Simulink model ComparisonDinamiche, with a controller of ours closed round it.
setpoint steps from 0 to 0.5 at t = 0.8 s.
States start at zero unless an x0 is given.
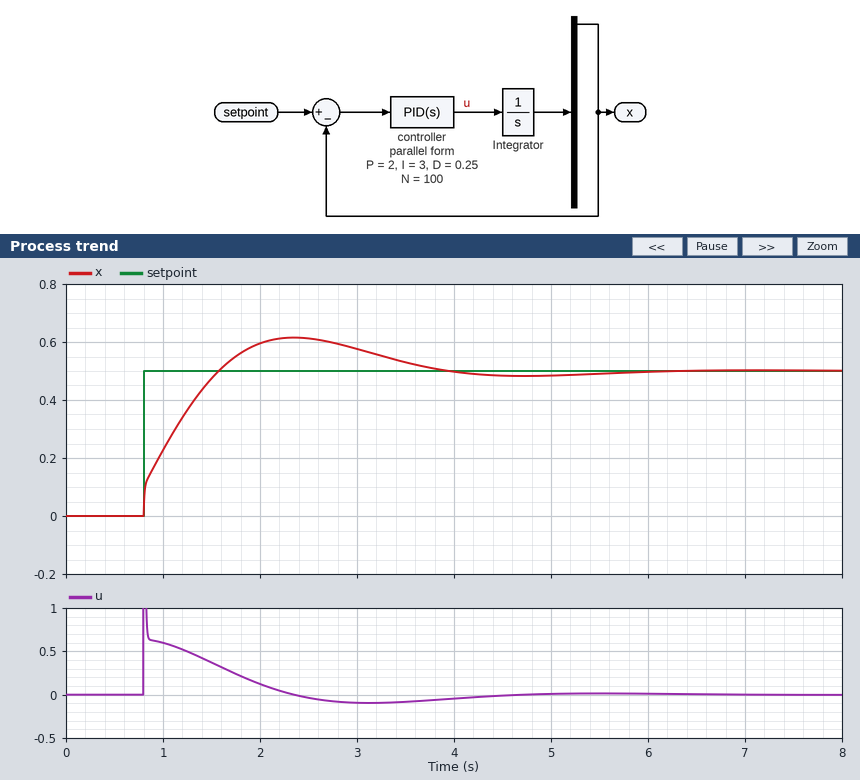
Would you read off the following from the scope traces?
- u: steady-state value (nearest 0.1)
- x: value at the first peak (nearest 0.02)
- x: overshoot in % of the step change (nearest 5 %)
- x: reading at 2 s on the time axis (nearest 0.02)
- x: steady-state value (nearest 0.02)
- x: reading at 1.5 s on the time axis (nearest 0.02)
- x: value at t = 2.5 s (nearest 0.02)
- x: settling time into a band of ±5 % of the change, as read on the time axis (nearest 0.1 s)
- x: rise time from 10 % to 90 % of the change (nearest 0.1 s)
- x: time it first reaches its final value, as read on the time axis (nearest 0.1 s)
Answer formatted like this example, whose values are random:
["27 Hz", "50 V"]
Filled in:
["0.0", "0.62", "25 %", "0.60", "0.50", "0.48", "0.62", "3.6 s", "0.6 s", "1.6 s"]
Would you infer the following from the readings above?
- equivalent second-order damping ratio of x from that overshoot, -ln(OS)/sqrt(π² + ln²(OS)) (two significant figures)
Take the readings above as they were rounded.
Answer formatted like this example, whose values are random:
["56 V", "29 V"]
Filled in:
["0.40"]
